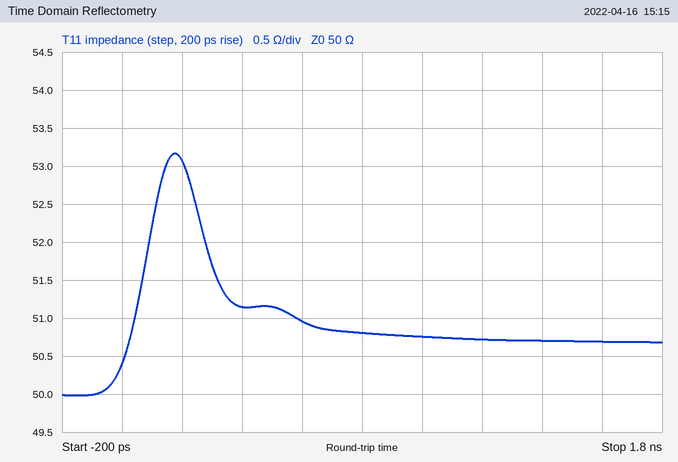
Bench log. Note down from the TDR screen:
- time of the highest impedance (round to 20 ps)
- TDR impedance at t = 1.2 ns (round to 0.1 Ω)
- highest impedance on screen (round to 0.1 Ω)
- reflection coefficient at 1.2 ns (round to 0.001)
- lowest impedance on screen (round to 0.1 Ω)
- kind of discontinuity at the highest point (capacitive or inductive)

180 ps
50.7 Ω
53.2 Ω
+0.007
50.0 Ω
inductive
